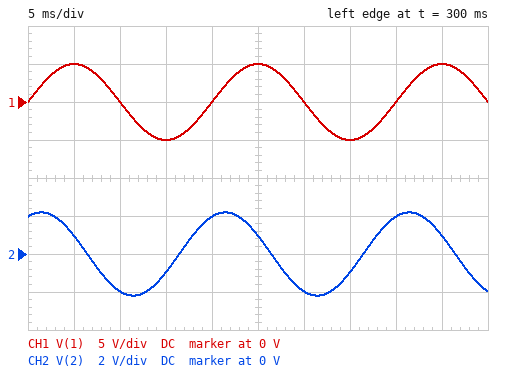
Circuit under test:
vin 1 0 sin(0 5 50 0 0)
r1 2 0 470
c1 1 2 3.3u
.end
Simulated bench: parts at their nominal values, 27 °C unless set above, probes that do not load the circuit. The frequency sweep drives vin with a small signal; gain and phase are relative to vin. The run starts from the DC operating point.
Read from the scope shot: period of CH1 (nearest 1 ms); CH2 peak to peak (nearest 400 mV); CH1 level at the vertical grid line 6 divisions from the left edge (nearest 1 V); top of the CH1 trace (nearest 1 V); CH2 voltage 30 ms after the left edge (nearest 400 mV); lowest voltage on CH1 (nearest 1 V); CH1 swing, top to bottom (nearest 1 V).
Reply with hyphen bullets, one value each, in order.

- 20 ms
- 4.4 V
- 0 V
- 5 V
- -2.0 V
- -5 V
- 10 V
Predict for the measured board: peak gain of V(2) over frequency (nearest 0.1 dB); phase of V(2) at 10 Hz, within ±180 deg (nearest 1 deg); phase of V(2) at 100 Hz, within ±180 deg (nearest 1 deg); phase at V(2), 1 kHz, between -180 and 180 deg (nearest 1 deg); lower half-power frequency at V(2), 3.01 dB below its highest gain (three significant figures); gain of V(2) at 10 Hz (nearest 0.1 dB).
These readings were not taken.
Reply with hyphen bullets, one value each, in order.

- 0 dB
- 84 deg
- 46 deg
- 6 deg
- 103 Hz
- -20.3 dB
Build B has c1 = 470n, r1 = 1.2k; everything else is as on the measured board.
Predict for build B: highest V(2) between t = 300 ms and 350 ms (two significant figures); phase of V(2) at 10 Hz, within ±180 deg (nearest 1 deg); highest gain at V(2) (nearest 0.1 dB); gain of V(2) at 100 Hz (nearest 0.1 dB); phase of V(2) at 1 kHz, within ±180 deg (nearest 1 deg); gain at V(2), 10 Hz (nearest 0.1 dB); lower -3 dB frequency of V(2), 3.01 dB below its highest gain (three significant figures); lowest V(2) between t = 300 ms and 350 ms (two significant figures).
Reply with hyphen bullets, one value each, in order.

- 870 mV
- 88 deg
- 0 dB
- -9.5 dB
- 16 deg
- -29.0 dB
- 282 Hz
- -870 mV
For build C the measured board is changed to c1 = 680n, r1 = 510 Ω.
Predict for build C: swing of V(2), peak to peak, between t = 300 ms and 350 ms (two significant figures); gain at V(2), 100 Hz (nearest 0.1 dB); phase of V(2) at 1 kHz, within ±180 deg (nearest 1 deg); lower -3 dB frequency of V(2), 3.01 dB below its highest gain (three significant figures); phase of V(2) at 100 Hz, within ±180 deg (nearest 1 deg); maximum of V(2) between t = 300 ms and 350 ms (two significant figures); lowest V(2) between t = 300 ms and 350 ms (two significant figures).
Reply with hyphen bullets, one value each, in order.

- 1.1 V
- -13.4 dB
- 25 deg
- 459 Hz
- 78 deg
- 540 mV
- -540 mV
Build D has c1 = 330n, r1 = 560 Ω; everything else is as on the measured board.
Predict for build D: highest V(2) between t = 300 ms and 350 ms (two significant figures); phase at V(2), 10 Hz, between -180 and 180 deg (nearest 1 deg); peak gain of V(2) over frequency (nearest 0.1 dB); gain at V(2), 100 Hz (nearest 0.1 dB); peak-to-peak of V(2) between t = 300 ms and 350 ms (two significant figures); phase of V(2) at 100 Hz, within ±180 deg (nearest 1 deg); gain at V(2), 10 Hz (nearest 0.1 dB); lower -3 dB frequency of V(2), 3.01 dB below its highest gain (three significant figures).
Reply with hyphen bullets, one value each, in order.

- 290 mV
- 89 deg
- 0 dB
- -18.8 dB
- 580 mV
- 83 deg
- -38.7 dB
- 861 Hz
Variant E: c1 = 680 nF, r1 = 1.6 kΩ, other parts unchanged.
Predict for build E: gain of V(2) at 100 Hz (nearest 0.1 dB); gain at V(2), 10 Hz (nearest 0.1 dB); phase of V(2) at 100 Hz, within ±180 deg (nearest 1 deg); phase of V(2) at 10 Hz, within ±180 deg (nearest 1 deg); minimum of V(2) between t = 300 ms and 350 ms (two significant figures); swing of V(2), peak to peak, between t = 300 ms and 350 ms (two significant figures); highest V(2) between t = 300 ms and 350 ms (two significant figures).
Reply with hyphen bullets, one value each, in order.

- -5.0 dB
- -23.3 dB
- 56 deg
- 86 deg
- -1.6 V
- 3.2 V
- 1.6 V
